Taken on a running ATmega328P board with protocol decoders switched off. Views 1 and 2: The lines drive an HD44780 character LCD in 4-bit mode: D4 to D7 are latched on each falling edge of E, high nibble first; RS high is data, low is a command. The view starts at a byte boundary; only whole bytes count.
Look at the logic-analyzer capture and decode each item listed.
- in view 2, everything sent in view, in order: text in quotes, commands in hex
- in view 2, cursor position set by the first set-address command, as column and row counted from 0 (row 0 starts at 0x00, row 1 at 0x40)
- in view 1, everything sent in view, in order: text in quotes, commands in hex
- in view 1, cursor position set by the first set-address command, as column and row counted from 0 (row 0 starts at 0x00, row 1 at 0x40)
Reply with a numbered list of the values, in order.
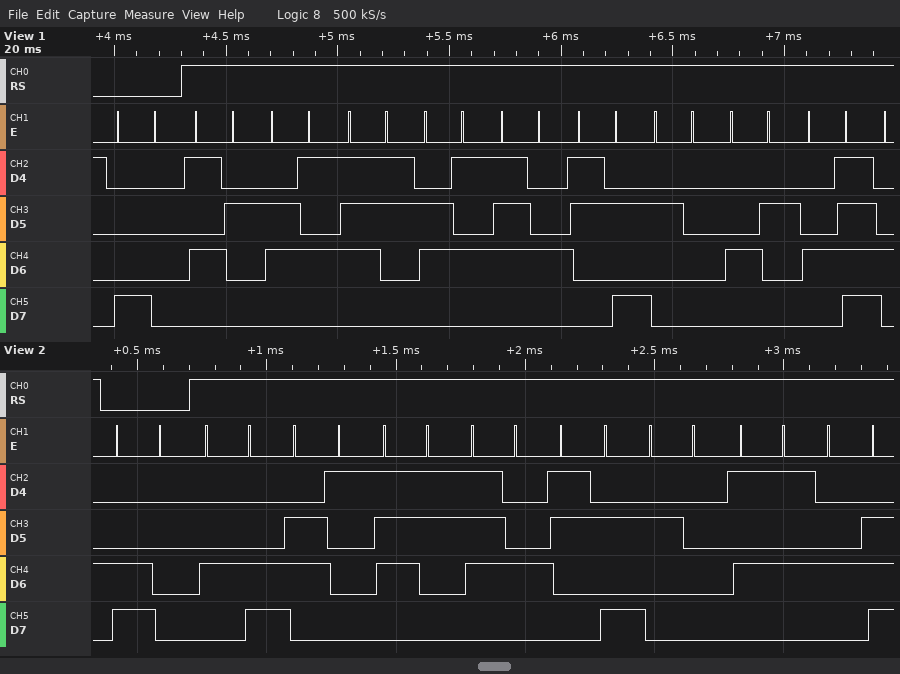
1. 0xC0 "Last: UN"
2. column 0, row 1
3. 0x80 "Reset: BO"
4. column 0, row 0
